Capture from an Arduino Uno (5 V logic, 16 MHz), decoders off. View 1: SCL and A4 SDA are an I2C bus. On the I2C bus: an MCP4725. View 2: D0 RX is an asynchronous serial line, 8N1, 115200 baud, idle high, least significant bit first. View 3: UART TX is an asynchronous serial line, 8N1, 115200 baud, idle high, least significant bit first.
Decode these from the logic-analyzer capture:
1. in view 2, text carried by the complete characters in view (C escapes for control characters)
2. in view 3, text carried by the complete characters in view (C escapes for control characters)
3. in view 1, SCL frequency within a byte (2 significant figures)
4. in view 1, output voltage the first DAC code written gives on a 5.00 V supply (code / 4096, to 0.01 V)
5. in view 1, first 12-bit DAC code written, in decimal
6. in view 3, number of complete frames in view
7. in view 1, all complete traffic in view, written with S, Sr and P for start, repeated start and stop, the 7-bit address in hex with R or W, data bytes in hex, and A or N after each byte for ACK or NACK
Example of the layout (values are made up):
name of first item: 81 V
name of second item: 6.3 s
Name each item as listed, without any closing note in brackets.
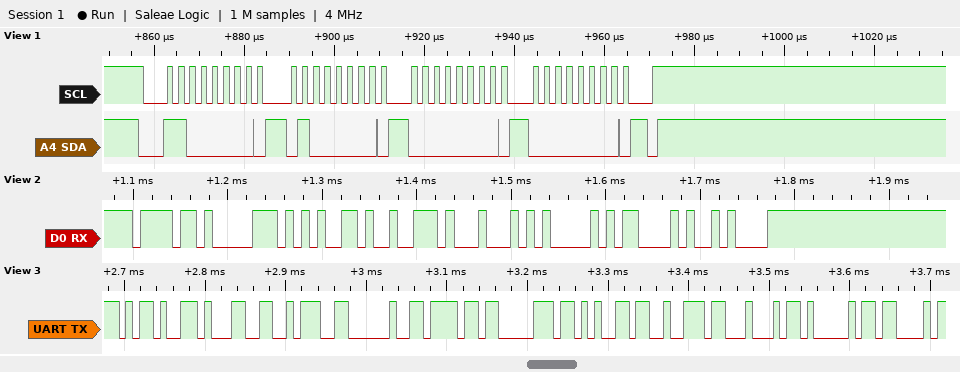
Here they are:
in view 2, text carried by the complete characters in view: "operDAC\n"
in view 3, text carried by the complete characters in view: "-1: operDAC"
in view 1, SCL frequency within a byte: 400 kHz
in view 1, output voltage the first DAC code written gives on a 5.00 V supply: 0.00 V
in view 1, first 12-bit DAC code written, in decimal: 0
in view 3, number of complete frames in view: 11
in view 1, all complete traffic in view, written with S, Sr and P for start, repeated start and stop, the 7-bit address in hex with R or W, data bytes in hex, and A or N after each byte for ACK or NACK: S 60W A 40 A 00 A 00 A P
